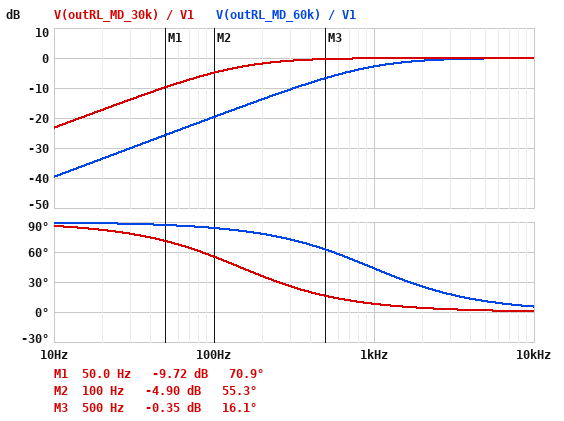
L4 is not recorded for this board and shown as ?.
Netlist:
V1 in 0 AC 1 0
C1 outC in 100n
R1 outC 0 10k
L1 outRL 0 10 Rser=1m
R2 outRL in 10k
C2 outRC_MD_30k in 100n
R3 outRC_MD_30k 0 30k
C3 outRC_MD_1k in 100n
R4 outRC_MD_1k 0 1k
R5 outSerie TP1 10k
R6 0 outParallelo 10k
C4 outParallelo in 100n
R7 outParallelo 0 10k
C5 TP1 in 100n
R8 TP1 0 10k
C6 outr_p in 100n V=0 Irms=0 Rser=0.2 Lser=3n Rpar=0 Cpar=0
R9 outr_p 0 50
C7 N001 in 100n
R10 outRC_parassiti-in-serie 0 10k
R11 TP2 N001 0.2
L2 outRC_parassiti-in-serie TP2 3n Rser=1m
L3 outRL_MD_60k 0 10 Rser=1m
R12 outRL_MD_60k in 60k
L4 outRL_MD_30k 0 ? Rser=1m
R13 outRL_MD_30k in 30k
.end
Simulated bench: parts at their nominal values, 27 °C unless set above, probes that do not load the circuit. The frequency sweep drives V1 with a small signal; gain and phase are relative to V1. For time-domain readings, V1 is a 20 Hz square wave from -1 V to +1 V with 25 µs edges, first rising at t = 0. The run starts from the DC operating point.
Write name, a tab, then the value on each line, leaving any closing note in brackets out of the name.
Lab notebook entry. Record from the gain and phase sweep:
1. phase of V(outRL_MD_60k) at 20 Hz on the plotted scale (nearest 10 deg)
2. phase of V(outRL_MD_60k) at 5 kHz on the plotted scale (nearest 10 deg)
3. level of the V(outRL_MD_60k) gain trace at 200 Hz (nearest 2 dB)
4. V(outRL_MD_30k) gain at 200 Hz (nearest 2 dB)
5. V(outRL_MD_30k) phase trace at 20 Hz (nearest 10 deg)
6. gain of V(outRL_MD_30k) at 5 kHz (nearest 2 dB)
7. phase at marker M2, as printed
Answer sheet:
phase of V(outRL_MD_60k) at 20 Hz on the plotted scale	90 deg
phase of V(outRL_MD_60k) at 5 kHz on the plotted scale	10 deg
level of the V(outRL_MD_60k) gain trace at 200 Hz	-14 dB
V(outRL_MD_30k) gain at 200 Hz	-2 dB
V(outRL_MD_30k) phase trace at 20 Hz	80 deg
gain of V(outRL_MD_30k) at 5 kHz	0 dB
phase at marker M2, as printed	55.3 deg
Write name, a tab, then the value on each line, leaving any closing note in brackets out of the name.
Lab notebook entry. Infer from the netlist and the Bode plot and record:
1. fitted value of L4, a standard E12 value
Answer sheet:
fitted value of L4, a standard E12 value	33 H
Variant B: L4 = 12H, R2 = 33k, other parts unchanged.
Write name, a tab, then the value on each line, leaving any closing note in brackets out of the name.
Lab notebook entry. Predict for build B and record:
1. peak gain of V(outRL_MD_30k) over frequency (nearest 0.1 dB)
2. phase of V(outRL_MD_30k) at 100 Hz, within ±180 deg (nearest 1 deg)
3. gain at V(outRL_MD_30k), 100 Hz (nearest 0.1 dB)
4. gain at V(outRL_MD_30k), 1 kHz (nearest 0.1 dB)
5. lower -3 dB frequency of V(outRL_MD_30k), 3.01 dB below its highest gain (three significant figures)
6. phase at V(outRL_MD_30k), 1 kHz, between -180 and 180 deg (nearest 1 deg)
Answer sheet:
peak gain of V(outRL_MD_30k) over frequency	0 dB
phase of V(outRL_MD_30k) at 100 Hz, within ±180 deg	76 deg
gain at V(outRL_MD_30k), 100 Hz	-12.3 dB
gain at V(outRL_MD_30k), 1 kHz	-0.6 dB
lower -3 dB frequency of V(outRL_MD_30k), 3.01 dB below its highest gain	398 Hz
phase at V(outRL_MD_30k), 1 kHz, between -180 and 180 deg	22 deg
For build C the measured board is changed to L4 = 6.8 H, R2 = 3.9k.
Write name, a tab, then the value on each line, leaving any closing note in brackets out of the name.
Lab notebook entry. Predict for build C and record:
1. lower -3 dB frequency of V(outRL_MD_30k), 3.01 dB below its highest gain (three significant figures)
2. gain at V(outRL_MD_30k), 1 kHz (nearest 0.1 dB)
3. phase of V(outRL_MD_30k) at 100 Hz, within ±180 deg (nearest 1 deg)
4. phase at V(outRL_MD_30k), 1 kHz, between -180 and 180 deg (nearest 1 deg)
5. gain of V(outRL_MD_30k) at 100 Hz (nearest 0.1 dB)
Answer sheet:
lower -3 dB frequency of V(outRL_MD_30k), 3.01 dB below its highest gain	702 Hz
gain at V(outRL_MD_30k), 1 kHz	-1.7 dB
phase of V(outRL_MD_30k) at 100 Hz, within ±180 deg	82 deg
phase at V(outRL_MD_30k), 1 kHz, between -180 and 180 deg	35 deg
gain of V(outRL_MD_30k) at 100 Hz	-17.0 dB
